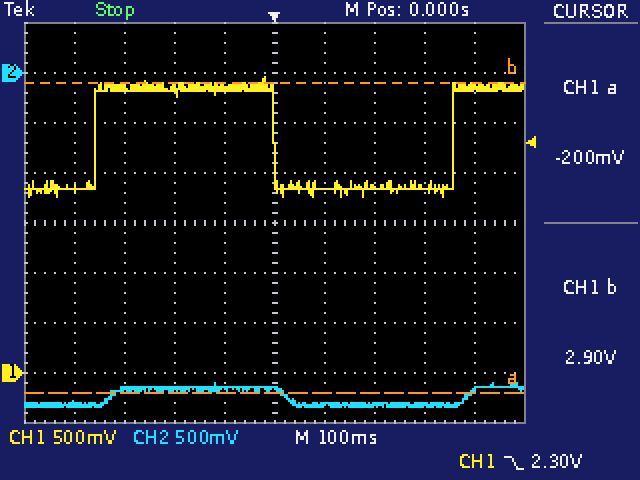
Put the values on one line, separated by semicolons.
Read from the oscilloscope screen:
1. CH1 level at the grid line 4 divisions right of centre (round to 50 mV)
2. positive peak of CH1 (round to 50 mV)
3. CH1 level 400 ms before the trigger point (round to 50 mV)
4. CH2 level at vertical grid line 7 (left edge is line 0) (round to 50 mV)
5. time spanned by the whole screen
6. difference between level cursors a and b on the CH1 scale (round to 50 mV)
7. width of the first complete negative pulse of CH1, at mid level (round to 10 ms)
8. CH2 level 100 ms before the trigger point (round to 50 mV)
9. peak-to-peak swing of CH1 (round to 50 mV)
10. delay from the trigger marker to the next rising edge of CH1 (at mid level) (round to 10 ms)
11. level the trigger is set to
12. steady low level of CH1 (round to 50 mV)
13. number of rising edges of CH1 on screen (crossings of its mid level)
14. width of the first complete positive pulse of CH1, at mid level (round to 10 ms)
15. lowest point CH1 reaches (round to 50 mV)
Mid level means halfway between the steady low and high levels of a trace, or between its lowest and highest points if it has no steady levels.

2.85 V; 2.95 V; 1.85 V; -3.30 V; 1 s; 3.10 V; 360 ms; -3.15 V; 1.20 V; 360 ms; 2.30 V; 1.85 V; 2; 360 ms; 1.75 V
